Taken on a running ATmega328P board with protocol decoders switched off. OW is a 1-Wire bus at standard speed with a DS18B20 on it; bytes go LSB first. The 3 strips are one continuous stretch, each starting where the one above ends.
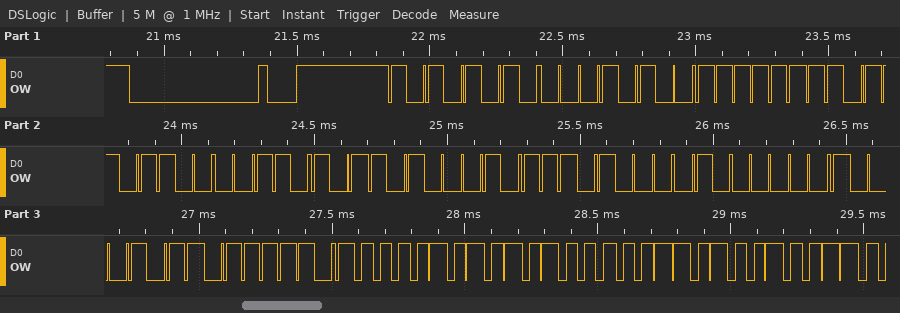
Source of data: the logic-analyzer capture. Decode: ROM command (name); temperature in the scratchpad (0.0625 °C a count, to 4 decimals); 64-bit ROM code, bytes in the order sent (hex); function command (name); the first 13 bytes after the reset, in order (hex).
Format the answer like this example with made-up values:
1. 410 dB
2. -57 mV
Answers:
1. Match ROM
2. 85.0000 °C
3. 28 FF 36 AC 45 17 02 D1
4. Read Scratchpad
5. 55 28 FF 36 AC 45 17 02 D1 BE 50 05 4B
